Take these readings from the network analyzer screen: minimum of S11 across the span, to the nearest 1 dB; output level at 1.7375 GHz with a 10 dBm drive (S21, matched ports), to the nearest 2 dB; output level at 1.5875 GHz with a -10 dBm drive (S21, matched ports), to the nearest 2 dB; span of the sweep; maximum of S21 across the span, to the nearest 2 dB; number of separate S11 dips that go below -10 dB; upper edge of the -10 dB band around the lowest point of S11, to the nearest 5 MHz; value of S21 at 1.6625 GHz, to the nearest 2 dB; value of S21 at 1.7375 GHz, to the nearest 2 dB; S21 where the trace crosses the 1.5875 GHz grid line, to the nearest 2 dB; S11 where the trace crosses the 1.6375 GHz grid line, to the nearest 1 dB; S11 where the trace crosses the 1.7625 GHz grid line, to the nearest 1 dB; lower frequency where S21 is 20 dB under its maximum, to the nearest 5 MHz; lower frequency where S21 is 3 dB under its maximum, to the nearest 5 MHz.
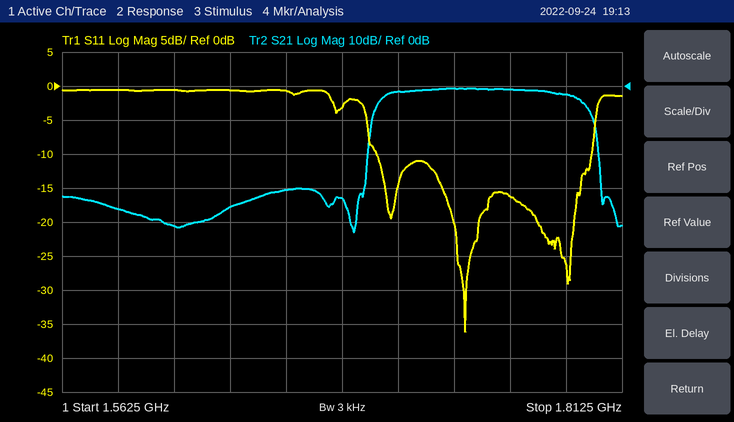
-36 dB
10 dBm
-46 dBm
250 MHz
0 dB
3
1.800 GHz
-30 dB
0 dB
-36 dB
-1 dB
-16 dB
1.700 GHz
1.705 GHz
